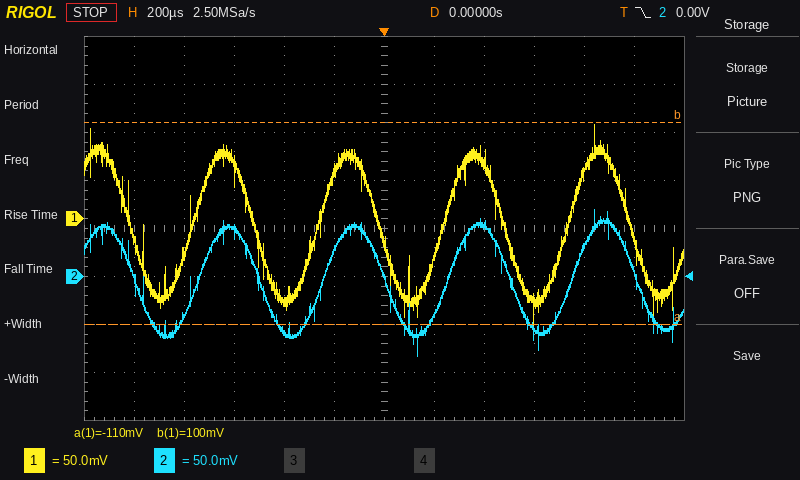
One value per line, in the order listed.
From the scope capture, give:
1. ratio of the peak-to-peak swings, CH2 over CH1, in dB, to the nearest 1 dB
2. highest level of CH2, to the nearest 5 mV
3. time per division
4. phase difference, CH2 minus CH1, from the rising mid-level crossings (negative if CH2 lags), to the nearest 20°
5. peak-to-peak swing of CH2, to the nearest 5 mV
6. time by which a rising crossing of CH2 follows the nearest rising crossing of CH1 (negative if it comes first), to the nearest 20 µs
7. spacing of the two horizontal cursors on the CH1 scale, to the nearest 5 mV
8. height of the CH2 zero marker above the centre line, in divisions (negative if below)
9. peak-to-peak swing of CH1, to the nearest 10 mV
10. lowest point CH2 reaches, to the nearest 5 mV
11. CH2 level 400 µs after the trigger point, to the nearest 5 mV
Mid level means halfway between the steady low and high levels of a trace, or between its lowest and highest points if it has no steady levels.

-3 dB
70 mV
200 µs
-20°
150 mV
+20 µs
210 mV
-1.0 div
210 mV
-80 mV
55 mV
